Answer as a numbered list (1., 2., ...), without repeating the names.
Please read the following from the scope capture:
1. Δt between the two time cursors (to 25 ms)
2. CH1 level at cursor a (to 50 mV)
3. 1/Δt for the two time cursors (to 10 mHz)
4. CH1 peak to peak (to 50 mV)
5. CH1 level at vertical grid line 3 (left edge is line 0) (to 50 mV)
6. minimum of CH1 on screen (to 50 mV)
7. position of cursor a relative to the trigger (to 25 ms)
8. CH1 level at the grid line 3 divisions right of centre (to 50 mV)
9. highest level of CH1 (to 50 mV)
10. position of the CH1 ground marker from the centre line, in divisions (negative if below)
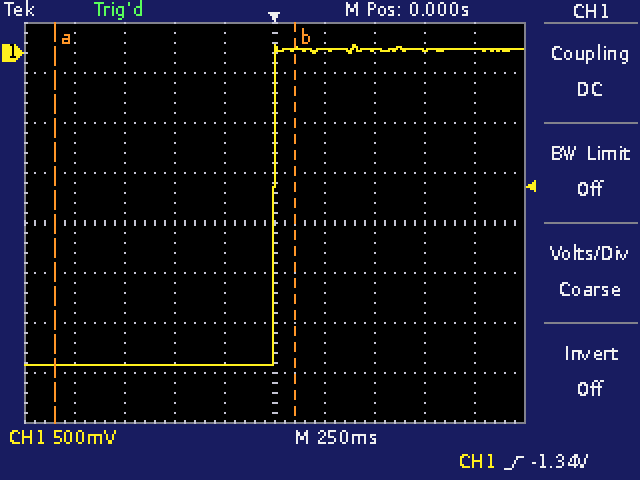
1. 1.200 s
2. -3.10 V
3. 830 mHz
4. 3.20 V
5. -3.10 V
6. -3.10 V
7. -1.100 s
8. 50 mV
9. 100 mV
10. +3.4 div
